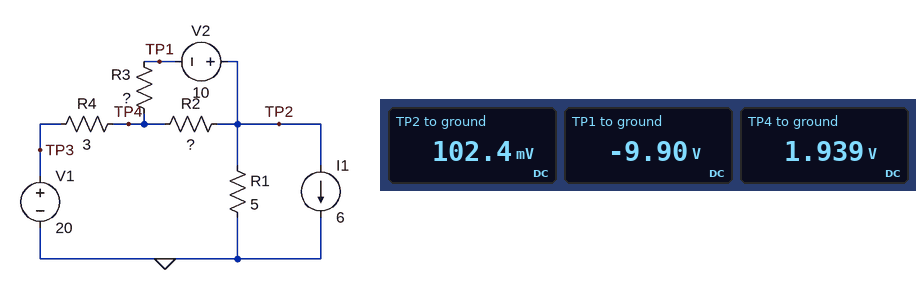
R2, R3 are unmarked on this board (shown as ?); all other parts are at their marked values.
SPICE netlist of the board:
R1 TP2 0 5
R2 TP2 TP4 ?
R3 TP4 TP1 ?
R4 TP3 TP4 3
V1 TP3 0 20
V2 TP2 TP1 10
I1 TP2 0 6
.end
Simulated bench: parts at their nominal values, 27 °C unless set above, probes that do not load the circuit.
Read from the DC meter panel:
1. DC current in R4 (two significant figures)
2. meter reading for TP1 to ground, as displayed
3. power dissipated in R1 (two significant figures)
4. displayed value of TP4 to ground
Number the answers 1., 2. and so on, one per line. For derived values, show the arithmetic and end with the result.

1. (20 V - 1.939 V) / 3 Ω = 6.0 A
2. -9.90 V
3. (102.4 mV)^2 / 5 Ω = 2.1 mW
4. 1.939 V
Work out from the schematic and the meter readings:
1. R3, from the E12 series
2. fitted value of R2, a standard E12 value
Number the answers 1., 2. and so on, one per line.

1. 5.6 Ω
2. 0.47 Ω
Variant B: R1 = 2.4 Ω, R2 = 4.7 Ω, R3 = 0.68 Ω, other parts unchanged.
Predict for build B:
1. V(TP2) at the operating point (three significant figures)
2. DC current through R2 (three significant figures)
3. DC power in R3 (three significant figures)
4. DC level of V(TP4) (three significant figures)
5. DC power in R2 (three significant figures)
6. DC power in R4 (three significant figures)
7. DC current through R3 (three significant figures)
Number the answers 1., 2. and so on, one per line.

1. 2.87 V
2. 949 mA
3. 45.1 W
4. -1.59 V
5. 4.23 W
6. 155 W
7. 8.15 A
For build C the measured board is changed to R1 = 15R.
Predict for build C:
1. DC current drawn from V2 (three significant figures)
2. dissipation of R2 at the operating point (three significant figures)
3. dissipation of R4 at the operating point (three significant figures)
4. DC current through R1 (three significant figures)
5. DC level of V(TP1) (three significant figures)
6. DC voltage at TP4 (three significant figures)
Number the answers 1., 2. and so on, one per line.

1. 2.11 A
2. 7.14 W
3. 108 W
4. 9.37 mA
5. -9.86 V
6. 1.97 V
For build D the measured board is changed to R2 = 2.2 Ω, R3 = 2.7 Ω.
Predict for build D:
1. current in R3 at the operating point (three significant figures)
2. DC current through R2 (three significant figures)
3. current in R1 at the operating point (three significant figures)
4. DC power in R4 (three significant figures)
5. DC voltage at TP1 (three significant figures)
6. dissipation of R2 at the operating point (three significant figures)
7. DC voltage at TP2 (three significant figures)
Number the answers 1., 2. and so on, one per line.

1. 4.70 A
2. 1.22 A
3. 85.1 mA
4. 105 W
5. -10.4 V
6. 3.27 W
7. -425 mV
